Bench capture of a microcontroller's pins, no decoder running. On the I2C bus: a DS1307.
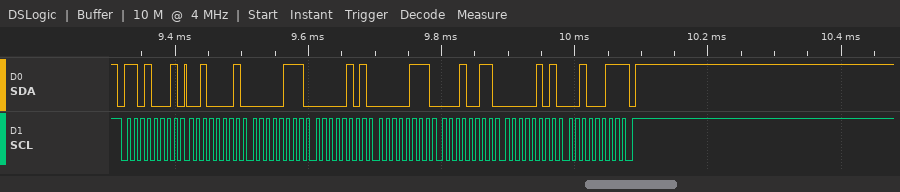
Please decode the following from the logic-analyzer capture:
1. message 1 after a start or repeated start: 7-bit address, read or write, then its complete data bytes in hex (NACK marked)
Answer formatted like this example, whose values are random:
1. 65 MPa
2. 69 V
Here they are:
1. 0x68 read: 21 07 05 07 13 05 23 NACK
